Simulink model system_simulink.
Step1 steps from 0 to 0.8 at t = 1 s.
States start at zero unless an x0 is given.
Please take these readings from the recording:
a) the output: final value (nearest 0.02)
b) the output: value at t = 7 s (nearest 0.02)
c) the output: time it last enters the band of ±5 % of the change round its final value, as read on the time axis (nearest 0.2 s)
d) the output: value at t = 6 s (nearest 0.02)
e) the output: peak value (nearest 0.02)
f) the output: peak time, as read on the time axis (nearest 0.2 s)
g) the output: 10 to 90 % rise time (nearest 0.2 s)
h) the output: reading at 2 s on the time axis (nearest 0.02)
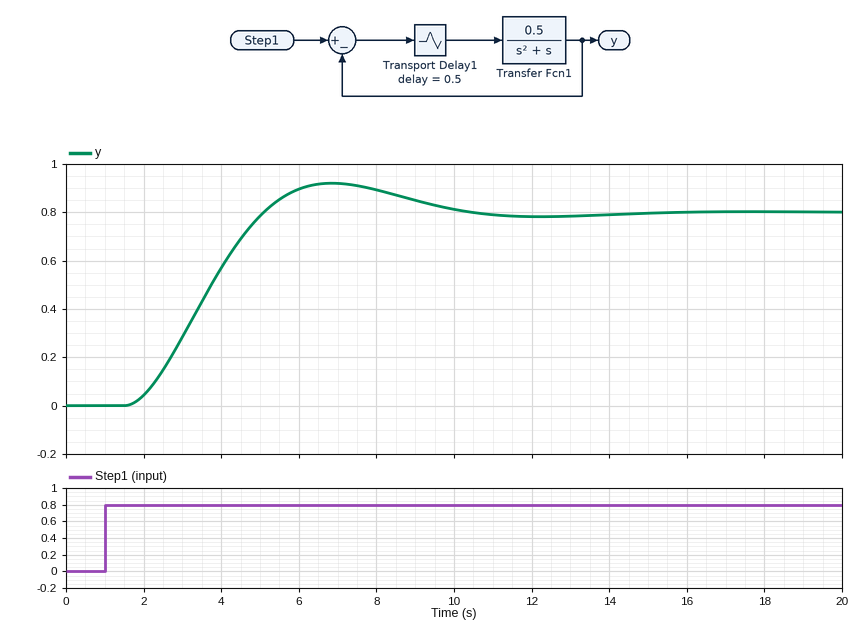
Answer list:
0.80
0.92
9.2 s
0.90
0.92
6.8 s
2.4 s
0.04
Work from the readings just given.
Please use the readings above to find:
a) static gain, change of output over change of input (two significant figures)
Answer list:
1.0
